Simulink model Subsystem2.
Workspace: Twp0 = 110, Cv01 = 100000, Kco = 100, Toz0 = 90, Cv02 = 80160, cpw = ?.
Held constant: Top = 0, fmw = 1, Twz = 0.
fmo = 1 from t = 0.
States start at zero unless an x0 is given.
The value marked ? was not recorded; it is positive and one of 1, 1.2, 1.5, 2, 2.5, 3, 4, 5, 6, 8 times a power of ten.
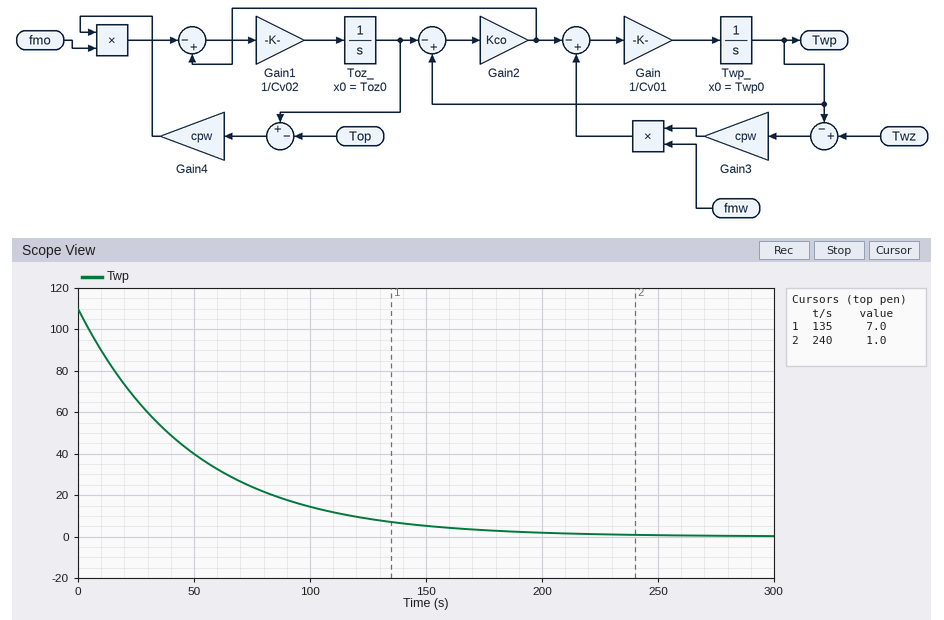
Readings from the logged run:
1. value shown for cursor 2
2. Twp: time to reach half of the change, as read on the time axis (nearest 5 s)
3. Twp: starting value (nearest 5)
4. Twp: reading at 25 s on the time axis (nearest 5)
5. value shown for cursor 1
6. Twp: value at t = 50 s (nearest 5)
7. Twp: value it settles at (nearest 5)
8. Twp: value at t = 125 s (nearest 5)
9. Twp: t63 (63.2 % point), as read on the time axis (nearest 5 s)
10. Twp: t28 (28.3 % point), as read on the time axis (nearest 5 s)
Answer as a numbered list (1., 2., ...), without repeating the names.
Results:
1. 1.0
2. 35 s
3. 110
4. 65
5. 7.0
6. 40
7. 0
8. 10
9. 50 s
10. 15 s
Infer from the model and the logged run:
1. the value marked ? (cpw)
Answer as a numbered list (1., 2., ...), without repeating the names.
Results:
1. 2000
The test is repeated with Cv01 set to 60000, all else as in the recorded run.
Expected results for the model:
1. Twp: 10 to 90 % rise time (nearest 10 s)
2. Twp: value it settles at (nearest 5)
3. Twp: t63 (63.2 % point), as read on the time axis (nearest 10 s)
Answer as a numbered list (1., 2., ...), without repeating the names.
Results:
1. 70 s
2. 0
3. 30 s
